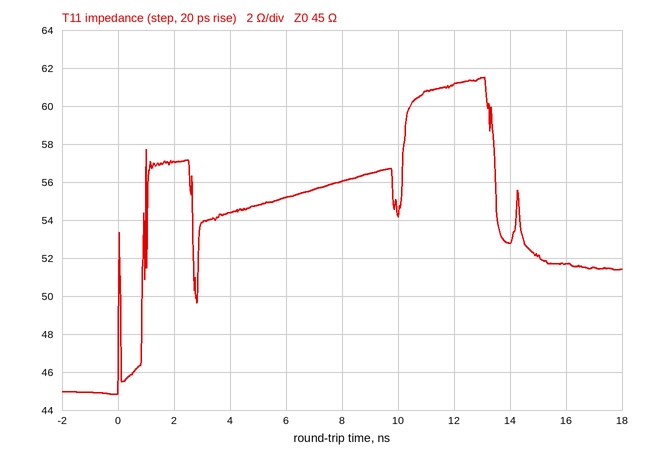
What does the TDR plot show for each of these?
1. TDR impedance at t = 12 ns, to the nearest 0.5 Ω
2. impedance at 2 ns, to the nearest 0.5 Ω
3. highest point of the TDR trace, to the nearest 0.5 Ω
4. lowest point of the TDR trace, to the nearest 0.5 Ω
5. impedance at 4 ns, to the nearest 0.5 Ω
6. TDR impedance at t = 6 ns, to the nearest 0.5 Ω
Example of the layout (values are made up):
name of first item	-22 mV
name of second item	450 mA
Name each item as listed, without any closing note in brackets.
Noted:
TDR impedance at t = 12 ns, to the nearest 0.5 Ω	61.0 Ω
impedance at 2 ns, to the nearest 0.5 Ω	57.0 Ω
highest point of the TDR trace, to the nearest 0.5 Ω	61.5 Ω
lowest point of the TDR trace, to the nearest 0.5 Ω	45.0 Ω
impedance at 4 ns, to the nearest 0.5 Ω	54.5 Ω
TDR impedance at t = 6 ns, to the nearest 0.5 Ω	55.0 Ω
